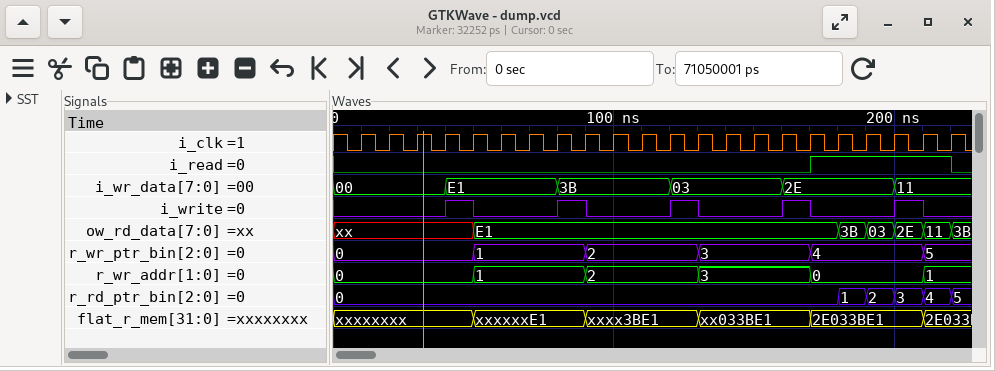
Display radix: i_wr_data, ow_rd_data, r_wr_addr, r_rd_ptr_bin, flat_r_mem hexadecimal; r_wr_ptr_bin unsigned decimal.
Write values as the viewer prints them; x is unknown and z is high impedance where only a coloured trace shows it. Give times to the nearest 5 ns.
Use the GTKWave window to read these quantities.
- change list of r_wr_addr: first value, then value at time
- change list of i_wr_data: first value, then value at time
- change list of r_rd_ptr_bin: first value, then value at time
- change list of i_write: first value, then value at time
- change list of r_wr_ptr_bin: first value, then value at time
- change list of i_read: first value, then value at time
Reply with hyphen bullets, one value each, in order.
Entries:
- 0, 1 at 50 ns, 2 at 90 ns, 3 at 130 ns, 0 at 170 ns, 1 at 210 ns
- 00, E1 at 40 ns, 3B at 80 ns, 03 at 120 ns, 2E at 160 ns, 11 at 200 ns
- 0, 1 at 180 ns, 2 at 190 ns, 3 at 200 ns, 4 at 210 ns, 5 at 220 ns
- 0, 1 at 40 ns, 0 at 50 ns, 1 at 80 ns, 0 at 90 ns, 1 at 120 ns, 0 at 130 ns, 1 at 160 ns, 0 at 170 ns, 1 at 200 ns, 0 at 210 ns
- 0, 1 at 50 ns, 2 at 90 ns, 3 at 130 ns, 4 at 170 ns, 5 at 210 ns
- 0, 1 at 170 ns, 0 at 220 ns
